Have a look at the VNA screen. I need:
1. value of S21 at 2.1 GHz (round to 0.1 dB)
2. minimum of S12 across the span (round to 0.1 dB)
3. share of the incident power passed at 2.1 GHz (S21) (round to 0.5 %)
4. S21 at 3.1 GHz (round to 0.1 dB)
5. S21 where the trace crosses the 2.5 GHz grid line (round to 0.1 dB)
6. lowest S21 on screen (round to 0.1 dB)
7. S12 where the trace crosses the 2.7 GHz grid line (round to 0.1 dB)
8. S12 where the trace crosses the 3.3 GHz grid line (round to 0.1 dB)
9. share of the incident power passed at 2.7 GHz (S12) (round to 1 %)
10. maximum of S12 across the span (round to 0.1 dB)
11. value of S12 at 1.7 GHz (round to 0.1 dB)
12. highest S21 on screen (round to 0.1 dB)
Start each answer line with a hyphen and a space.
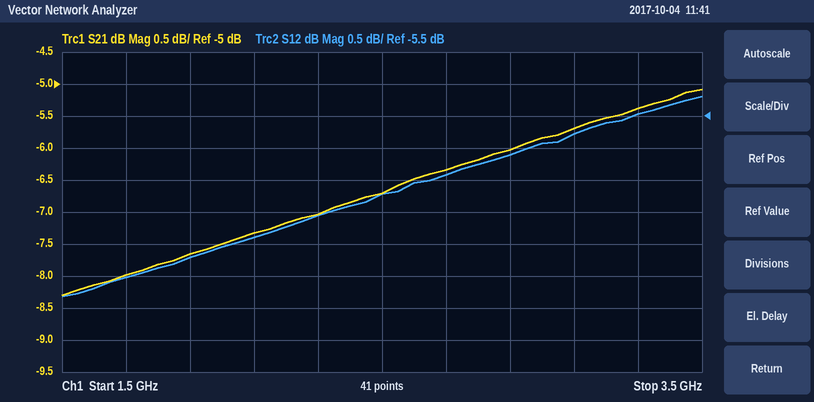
- -7.3 dB
- -8.3 dB
- 18.5 %
- -5.7 dB
- -6.7 dB
- -8.3 dB
- -6.4 dB
- -5.5 dB
- 23 %
- -5.2 dB
- -8.0 dB
- -5.1 dB
